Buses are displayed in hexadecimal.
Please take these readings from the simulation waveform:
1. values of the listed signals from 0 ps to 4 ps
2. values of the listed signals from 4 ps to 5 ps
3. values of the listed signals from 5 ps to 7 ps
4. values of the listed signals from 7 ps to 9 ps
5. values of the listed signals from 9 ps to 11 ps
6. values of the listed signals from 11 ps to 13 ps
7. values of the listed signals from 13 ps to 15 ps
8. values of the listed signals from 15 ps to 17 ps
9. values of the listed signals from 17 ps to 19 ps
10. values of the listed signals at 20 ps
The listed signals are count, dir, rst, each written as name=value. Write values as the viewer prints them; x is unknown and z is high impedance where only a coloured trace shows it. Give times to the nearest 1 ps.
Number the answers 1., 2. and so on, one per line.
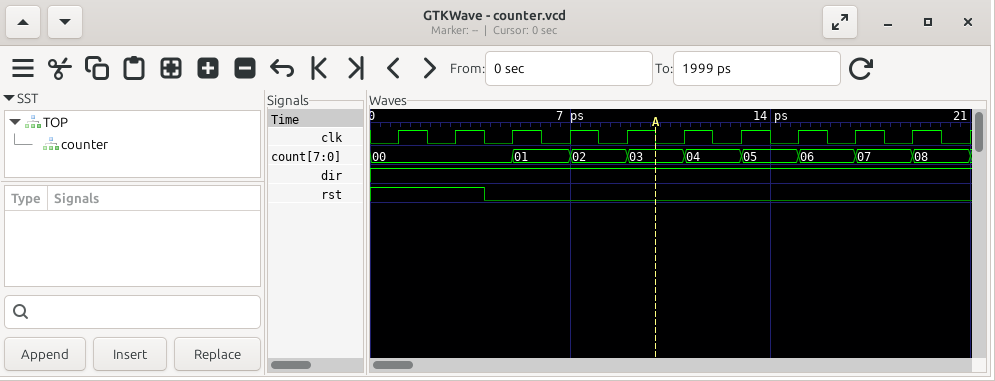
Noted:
1. count=00, dir=1, rst=1
2. count=00, dir=1, rst=0
3. count=01, dir=1, rst=0
4. count=02, dir=1, rst=0
5. count=03, dir=1, rst=0
6. count=04, dir=1, rst=0
7. count=05, dir=1, rst=0
8. count=06, dir=1, rst=0
9. count=07, dir=1, rst=0
10. count=08, dir=1, rst=0
